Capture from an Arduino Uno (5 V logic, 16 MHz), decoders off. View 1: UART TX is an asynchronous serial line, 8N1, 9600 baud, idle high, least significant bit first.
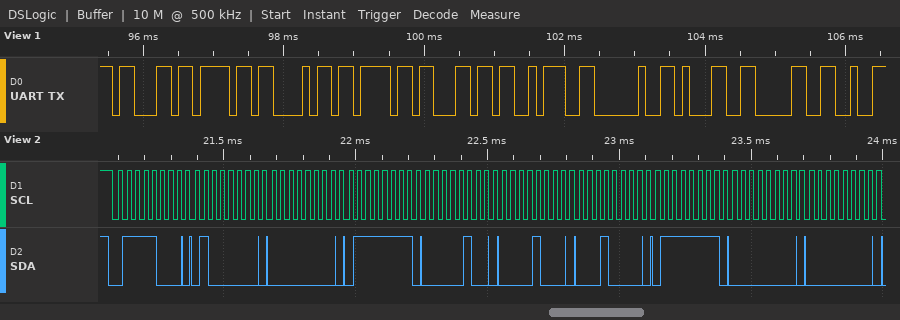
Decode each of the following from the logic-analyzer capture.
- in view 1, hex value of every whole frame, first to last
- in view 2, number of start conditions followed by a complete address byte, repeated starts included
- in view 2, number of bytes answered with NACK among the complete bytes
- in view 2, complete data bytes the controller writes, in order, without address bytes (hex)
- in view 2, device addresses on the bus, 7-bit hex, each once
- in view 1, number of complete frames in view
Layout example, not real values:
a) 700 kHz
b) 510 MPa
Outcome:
a) 63 6F 68 6F 6C 3A 20 31 30
b) 1
c) 0
d) 40 00 7F 04 08 10 7F 00 00
e) 0x3C
f) 9
